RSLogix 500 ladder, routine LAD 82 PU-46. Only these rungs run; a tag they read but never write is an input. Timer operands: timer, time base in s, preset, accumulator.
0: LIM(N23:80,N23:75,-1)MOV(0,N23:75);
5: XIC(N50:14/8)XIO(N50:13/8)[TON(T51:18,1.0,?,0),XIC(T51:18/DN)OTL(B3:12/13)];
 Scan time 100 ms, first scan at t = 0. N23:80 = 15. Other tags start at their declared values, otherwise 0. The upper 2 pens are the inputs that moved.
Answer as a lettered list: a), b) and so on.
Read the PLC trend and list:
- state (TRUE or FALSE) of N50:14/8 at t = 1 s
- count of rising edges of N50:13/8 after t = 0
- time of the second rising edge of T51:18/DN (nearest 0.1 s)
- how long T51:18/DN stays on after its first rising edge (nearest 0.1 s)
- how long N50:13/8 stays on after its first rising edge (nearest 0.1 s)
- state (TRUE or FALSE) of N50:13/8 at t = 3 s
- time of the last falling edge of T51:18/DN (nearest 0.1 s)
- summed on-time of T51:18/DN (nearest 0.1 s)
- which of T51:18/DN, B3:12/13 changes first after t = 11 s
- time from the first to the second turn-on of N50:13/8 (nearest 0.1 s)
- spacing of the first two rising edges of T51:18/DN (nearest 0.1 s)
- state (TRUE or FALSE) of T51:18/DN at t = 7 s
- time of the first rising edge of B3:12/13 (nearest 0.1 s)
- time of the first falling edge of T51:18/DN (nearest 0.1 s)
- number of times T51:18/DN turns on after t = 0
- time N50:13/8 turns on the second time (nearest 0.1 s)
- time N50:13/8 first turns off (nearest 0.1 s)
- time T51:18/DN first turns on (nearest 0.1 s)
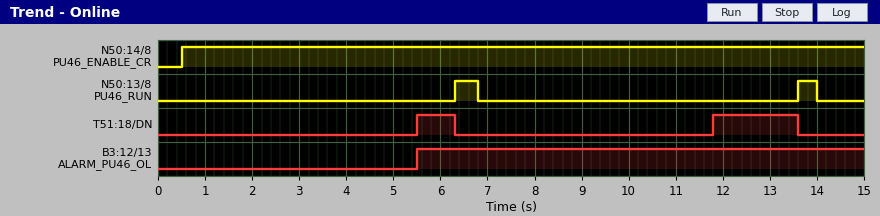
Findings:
a) TRUE
b) 2
c) 11.8 s
d) 0.8 s
e) 0.5 s
f) FALSE
g) 13.6 s
h) 2.6 s
i) T51:18/DN
j) 7.3 s
k) 6.3 s
l) FALSE
m) 5.5 s
n) 6.3 s
o) 2
p) 13.6 s
q) 6.8 s
r) 5.5 s
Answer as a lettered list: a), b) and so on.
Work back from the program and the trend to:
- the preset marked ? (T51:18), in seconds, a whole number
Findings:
a) 5 s
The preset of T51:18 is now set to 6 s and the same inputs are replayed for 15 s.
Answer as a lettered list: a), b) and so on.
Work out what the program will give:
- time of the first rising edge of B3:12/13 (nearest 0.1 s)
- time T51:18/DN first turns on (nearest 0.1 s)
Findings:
a) 12.8 s
b) 12.8 s
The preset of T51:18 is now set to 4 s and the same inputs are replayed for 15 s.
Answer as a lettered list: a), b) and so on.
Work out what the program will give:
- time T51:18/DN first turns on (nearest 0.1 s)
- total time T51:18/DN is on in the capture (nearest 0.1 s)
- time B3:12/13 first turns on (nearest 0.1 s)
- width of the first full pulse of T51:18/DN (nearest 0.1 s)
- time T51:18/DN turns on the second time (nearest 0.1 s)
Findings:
a) 4.5 s
b) 4.6 s
c) 4.5 s
d) 1.8 s
e) 10.8 s
